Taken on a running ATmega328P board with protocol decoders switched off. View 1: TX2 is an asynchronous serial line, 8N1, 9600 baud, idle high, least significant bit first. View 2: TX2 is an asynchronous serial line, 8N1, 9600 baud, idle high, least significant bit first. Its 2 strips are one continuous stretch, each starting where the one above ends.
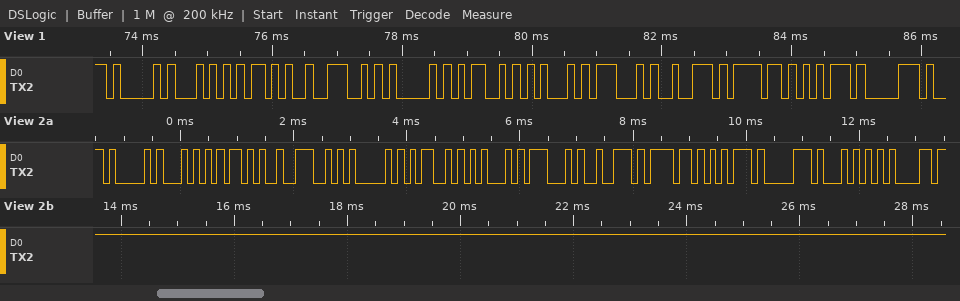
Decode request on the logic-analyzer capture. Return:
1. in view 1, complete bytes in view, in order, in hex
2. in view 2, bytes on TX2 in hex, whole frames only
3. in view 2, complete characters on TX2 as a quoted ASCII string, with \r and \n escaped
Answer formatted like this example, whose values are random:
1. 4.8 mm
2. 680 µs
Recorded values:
1. 41 54 2B 4E 41 4D 45 47 72 6F 75 70
2. 0x41 0x54 0x2B 0x4E 0x41 0x4D 0x45 0x47 0x72 0x6F 0x75 0x70 0x54 0x61
3. "AT+NAMEGroupTa"
